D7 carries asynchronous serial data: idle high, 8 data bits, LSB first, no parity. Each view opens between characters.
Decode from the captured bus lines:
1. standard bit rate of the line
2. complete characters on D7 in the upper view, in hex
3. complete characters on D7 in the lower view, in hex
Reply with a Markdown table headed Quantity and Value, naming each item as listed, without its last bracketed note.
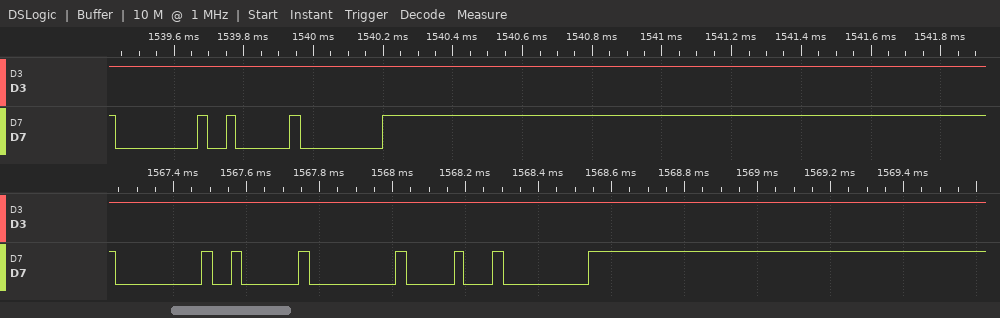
| Quantity | Value |
|---|---|
| standard bit rate of the line | 38400 baud |
| complete characters on D7 in the upper view, in hex | 00, 02, 00 |
| complete characters on D7 in the lower view, in hex | 00, 02, 00, 10, 00 |
